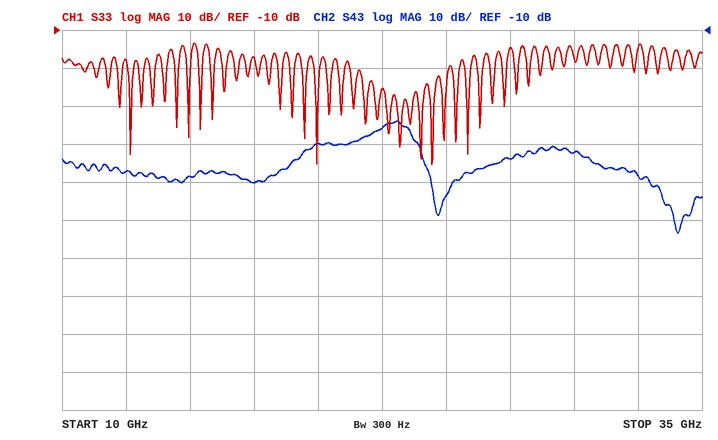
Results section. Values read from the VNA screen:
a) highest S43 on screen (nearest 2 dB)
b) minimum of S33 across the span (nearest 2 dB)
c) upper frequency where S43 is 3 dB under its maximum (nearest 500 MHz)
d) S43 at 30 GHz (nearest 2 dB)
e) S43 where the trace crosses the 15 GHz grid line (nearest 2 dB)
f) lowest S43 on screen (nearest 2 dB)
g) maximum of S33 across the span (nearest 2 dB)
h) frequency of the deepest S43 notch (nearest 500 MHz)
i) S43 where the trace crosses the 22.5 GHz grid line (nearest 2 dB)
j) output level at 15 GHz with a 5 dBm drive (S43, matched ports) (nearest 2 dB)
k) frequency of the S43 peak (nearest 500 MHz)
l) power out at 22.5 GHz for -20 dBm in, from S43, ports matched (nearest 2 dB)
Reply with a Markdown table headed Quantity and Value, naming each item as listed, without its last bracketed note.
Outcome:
| Quantity | Value |
|---|---|
| highest S43 on screen | -34 dB |
| minimum of S33 across the span | -46 dB |
| upper frequency where S43 is 3 dB under its maximum | 23.5 GHz |
| S43 at 30 GHz | -42 dB |
| S43 where the trace crosses the 15 GHz grid line | -48 dB |
| lowest S43 on screen | -64 dB |
| maximum of S33 across the span | -14 dB |
| frequency of the deepest S43 notch | 34.0 GHz |
| S43 where the trace crosses the 22.5 GHz grid line | -36 dB |
| output level at 15 GHz with a 5 dBm drive (S43, matched ports) | -44 dBm |
| frequency of the S43 peak | 23.0 GHz |
| power out at 22.5 GHz for -20 dBm in, from S43, ports matched | -56 dBm |
